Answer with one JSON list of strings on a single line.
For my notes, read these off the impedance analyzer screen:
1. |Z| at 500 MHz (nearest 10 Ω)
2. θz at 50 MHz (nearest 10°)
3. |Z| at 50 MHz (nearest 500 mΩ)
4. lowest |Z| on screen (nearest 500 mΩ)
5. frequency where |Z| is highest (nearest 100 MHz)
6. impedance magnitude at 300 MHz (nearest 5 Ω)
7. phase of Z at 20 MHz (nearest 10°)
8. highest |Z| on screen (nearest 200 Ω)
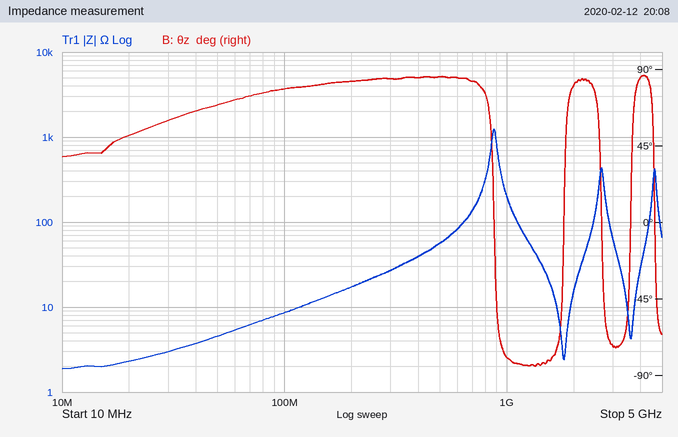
["60 Ω", "70°", "4.5 Ω", "2.0 Ω", "900 MHz", "25 Ω", "50°", "1.2 kΩ"]
